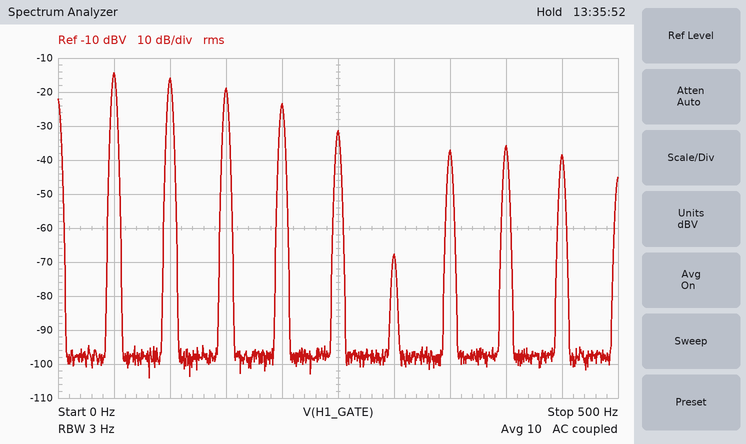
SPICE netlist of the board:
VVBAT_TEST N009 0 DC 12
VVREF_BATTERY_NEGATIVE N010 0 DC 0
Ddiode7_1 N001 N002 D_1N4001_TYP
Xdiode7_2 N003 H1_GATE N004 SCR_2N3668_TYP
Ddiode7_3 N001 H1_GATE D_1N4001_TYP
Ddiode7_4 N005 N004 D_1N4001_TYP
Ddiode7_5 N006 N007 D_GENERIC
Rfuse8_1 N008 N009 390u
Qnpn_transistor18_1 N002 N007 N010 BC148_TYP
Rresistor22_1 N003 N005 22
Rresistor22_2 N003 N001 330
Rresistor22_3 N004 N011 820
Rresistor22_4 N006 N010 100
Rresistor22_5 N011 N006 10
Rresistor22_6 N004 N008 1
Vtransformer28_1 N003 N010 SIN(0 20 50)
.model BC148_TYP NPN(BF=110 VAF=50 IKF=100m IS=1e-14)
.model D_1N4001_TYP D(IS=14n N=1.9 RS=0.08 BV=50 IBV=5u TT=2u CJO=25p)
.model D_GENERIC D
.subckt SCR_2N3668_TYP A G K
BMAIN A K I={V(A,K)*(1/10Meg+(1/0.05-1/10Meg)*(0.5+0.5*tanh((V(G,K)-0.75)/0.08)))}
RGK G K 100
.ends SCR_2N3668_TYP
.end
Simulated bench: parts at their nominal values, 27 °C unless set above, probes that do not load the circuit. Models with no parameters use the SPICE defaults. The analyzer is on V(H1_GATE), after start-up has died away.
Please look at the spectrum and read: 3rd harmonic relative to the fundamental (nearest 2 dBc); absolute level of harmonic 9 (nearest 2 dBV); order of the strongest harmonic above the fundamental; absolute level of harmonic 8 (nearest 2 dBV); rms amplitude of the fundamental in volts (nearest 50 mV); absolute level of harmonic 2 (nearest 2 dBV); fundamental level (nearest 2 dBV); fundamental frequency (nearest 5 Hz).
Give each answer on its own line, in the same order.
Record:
-4 dBc
-38 dBV
2
-36 dBV
200 mV
-16 dBV
-14 dBV
50 Hz
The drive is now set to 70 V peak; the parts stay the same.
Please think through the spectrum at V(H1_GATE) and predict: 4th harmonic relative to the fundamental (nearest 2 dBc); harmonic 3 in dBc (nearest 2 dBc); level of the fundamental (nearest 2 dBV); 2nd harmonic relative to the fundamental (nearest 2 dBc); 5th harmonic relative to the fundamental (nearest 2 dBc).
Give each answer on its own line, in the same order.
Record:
-18 dBc
-12 dBc
12 dBV
-12 dBc
-28 dBc
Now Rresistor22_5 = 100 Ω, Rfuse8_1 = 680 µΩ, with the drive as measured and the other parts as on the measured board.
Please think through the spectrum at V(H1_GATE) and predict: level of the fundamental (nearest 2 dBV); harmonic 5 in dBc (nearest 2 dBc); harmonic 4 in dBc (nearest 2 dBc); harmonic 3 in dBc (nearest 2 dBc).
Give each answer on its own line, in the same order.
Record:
-6 dBV
-60 dBc
-14 dBc
-6 dBc
